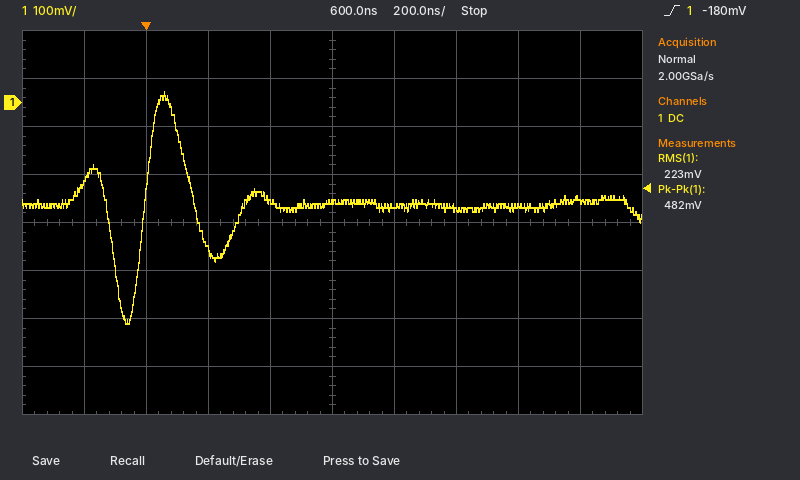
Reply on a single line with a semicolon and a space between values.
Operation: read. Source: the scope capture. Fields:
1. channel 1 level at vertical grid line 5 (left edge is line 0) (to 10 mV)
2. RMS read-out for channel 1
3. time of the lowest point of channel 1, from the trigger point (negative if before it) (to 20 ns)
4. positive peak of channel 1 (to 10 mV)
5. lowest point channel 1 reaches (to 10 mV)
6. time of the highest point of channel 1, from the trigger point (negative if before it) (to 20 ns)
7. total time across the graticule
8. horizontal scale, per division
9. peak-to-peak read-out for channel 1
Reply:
-210 mV; 223 mV; -60 ns; 20 mV; -460 mV; +60 ns; 2 µs; 200 ns; 482 mV
